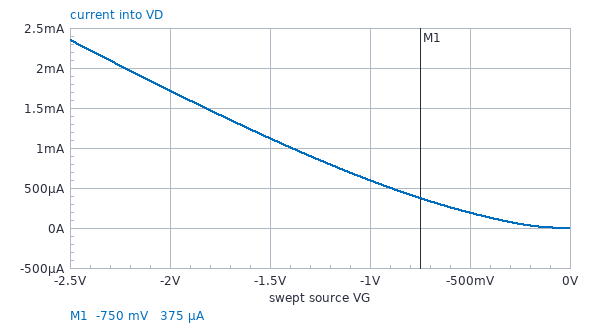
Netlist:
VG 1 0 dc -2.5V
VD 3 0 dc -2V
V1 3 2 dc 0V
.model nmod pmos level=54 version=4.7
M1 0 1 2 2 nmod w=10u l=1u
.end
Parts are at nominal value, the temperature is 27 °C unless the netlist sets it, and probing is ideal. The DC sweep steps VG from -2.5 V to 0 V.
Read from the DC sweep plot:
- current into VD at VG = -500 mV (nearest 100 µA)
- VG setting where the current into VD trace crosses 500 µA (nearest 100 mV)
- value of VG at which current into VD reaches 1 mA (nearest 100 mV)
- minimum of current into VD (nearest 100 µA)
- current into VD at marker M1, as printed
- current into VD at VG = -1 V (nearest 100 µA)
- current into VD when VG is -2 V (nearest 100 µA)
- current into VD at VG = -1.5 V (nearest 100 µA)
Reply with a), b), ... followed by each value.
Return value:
a) 200 µA
b) -900 mV
c) -1.4 V
d) 0 A
e) 375 µA
f) 600 µA
g) 1.7 mA
h) 1.1 mA
